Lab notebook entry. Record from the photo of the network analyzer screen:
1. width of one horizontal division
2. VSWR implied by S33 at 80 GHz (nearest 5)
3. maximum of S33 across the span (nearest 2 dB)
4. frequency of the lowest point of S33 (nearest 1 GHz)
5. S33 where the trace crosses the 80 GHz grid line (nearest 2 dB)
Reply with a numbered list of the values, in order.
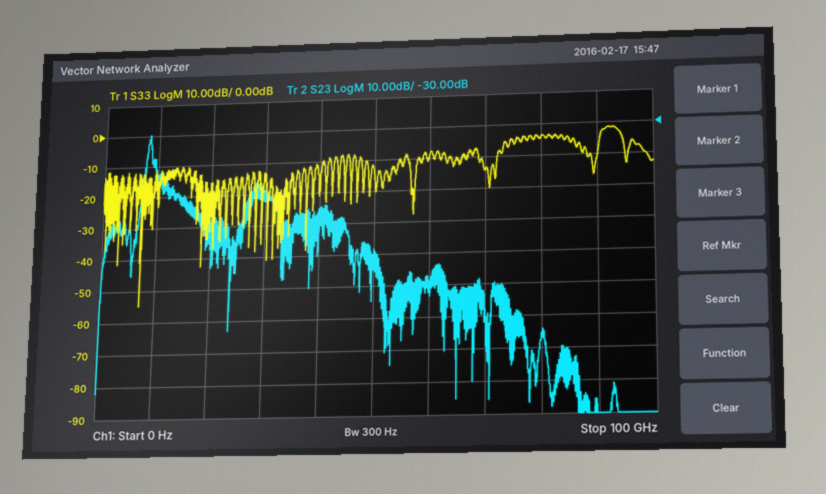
1. 10 GHz
2. 5
3. -2 dB
4. 7 GHz
5. -4 dB
